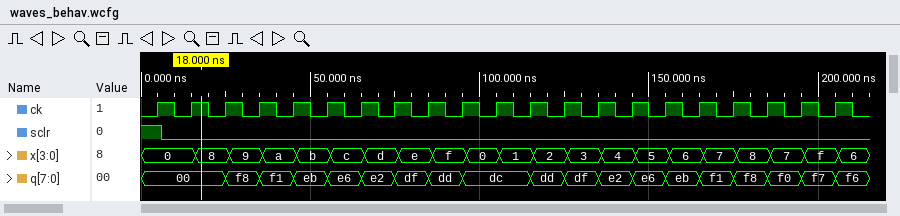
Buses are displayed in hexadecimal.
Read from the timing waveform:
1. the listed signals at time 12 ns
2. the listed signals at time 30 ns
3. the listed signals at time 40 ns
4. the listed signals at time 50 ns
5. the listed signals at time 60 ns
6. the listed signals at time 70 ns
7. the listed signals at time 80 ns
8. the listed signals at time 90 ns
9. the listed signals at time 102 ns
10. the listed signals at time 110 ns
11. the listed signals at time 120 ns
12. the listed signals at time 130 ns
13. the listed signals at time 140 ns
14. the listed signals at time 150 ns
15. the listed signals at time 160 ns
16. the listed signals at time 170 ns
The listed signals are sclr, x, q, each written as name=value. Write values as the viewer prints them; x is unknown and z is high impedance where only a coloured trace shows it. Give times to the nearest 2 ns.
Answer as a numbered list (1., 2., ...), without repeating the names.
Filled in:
1. sclr=0, x=0, q=00
2. sclr=0, x=9, q=f8
3. sclr=0, x=a, q=f1
4. sclr=0, x=b, q=eb
5. sclr=0, x=c, q=e6
6. sclr=0, x=d, q=e2
7. sclr=0, x=e, q=df
8. sclr=0, x=f, q=dd
9. sclr=0, x=0, q=dc
10. sclr=0, x=1, q=dc
11. sclr=0, x=2, q=dd
12. sclr=0, x=3, q=df
13. sclr=0, x=4, q=e2
14. sclr=0, x=5, q=e6
15. sclr=0, x=6, q=eb
16. sclr=0, x=7, q=f1
